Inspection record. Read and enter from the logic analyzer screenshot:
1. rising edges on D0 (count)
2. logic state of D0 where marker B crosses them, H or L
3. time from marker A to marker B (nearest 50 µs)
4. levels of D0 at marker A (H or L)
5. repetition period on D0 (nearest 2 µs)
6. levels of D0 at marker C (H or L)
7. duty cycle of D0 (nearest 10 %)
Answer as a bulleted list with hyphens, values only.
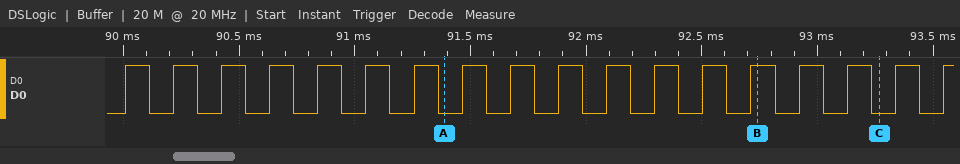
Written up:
- 18
- D0=H
- 1350 µs
- D0=L
- 208 µs
- D0=L
- 50 %
